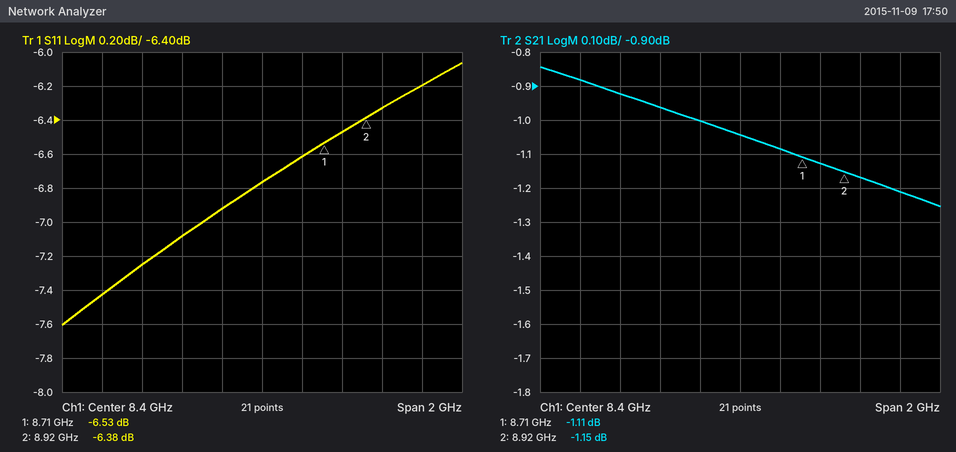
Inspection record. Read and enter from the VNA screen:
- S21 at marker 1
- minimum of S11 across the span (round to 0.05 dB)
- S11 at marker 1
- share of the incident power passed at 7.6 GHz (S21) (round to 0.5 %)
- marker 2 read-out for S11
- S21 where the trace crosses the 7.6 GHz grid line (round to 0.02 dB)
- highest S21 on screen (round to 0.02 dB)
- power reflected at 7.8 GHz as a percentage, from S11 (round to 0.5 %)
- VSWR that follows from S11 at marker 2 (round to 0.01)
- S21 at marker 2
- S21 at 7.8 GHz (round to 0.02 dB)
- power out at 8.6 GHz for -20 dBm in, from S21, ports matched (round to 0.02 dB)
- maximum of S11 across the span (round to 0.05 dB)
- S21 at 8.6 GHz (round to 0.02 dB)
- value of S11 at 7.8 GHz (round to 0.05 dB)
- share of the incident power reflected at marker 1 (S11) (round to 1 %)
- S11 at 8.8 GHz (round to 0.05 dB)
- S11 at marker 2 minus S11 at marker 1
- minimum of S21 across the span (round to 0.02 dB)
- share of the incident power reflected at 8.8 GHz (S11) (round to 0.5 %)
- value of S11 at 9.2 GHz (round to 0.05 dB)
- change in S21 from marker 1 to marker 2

-1.11 dB
-7.60 dB
-6.53 dB
81.5 %
-6.38 dB
-0.88 dB
-0.84 dB
19.0 %
2.84
-1.15 dB
-0.92 dB
-21.08 dBm
-6.05 dB
-1.08 dB
-7.25 dB
22 %
-6.45 dB
0.15 dB
-1.26 dB
22.5 %
-6.20 dB
-0.04 dB
